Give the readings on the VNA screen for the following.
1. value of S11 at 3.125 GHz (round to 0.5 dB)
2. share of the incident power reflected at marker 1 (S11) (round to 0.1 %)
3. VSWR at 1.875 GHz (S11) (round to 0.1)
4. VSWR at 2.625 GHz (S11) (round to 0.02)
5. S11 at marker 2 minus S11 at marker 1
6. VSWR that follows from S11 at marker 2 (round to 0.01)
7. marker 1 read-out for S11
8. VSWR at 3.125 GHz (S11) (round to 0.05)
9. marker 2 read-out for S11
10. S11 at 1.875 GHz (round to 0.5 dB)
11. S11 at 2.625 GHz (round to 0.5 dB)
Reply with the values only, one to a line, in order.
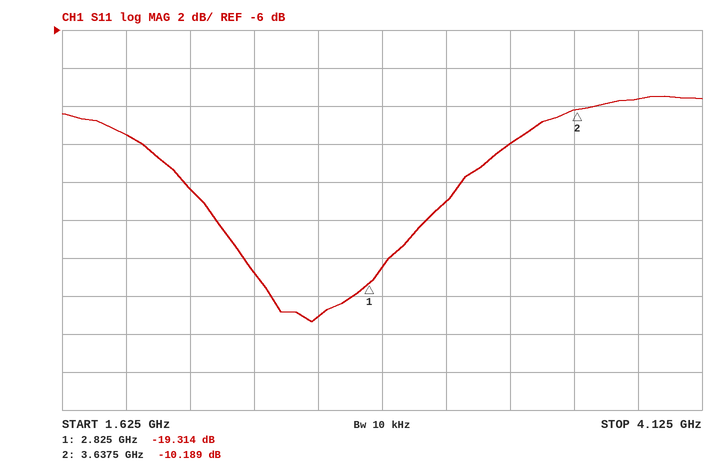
-15.0 dB
1.2 %
1.7
1.20
9.125 dB
1.90
-19.314 dB
1.45
-10.189 dB
-11.5 dB
-21.0 dB
